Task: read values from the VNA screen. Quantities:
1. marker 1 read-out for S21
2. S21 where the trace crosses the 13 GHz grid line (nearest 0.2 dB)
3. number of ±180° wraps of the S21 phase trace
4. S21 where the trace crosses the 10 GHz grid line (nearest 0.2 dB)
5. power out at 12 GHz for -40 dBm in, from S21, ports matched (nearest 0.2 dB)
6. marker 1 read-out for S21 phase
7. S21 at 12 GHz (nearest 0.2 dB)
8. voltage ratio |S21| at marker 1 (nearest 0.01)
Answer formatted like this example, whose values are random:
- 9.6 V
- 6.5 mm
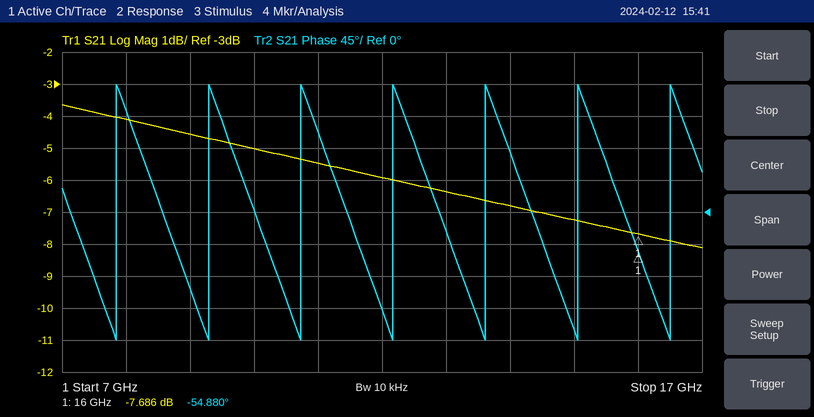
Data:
- -7.686 dB
- -6.4 dB
- 7
- -5.0 dB
- -46.0 dBm
- -54.880°
- -6.0 dB
- 0.41
